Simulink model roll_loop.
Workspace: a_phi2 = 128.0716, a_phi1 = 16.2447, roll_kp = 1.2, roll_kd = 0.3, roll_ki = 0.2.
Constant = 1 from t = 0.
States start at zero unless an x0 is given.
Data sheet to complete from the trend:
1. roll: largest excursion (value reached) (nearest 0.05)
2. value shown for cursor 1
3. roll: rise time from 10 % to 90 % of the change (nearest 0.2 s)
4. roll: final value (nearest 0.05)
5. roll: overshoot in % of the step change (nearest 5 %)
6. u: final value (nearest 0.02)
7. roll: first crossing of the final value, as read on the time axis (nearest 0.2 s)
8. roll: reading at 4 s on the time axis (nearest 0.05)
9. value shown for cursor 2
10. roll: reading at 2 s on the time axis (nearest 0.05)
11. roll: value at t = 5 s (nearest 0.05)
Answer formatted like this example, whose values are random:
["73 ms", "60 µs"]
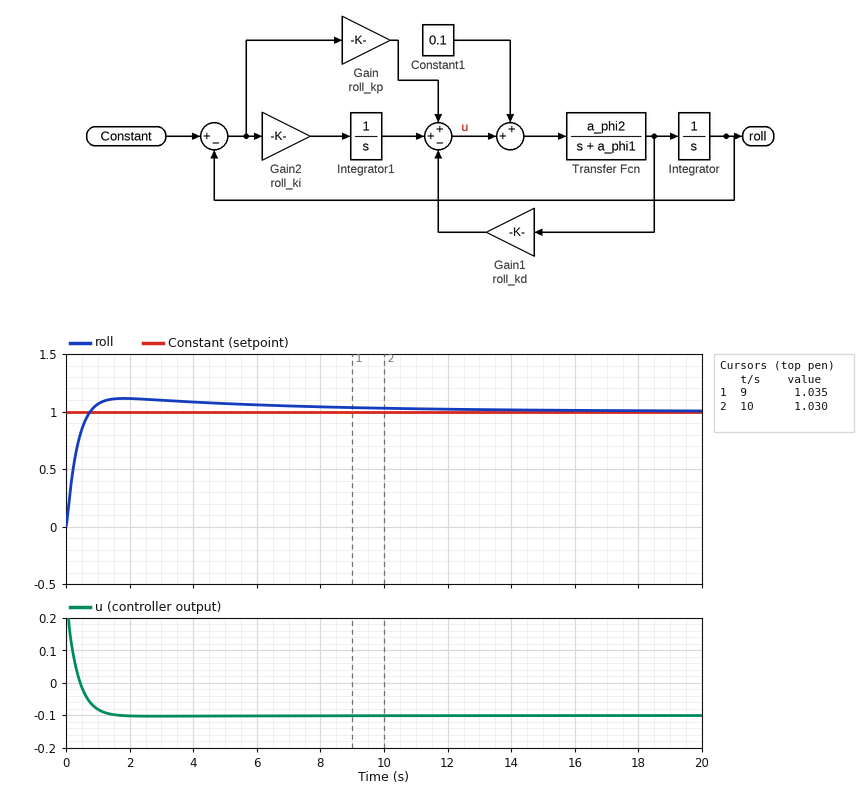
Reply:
["1.10", "1.035", "0.6 s", "1.00", "10 %", "-0.10", "0.8 s", "1.10", "1.030", "1.10", "1.05"]
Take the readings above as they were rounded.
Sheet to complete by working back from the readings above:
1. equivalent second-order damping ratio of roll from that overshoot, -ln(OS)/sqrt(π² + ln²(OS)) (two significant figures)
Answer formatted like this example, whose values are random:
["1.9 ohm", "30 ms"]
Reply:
["0.59"]
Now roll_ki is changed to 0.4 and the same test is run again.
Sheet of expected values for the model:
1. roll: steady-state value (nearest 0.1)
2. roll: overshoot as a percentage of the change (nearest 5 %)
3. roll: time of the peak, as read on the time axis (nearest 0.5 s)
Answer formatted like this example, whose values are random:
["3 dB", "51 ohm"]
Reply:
["1.0", "15 %", "1.5 s"]
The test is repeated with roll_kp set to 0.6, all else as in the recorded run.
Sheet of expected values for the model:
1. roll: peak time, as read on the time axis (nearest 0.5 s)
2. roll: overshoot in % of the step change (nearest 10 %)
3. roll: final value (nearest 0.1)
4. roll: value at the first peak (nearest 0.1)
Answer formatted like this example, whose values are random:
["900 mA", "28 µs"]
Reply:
["2.5 s", "20 %", "1.0", "1.2"]
